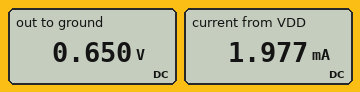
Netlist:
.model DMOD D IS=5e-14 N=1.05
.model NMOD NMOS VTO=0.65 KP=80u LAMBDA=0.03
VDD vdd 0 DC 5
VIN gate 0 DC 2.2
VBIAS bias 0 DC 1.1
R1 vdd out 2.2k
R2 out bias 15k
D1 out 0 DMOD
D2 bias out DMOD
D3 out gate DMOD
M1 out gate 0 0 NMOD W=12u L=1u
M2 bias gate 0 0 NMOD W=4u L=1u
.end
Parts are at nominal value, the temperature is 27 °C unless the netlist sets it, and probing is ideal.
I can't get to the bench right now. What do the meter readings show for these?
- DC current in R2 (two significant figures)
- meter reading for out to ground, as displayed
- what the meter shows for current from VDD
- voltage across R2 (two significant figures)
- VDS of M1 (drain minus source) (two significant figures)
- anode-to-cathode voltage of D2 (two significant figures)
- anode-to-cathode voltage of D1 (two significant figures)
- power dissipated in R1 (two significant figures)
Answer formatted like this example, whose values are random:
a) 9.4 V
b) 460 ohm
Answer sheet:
a) 30 µA
b) 0.650 V
c) 1.977 mA
d) 450 mV
e) 650 mV
f) 450 mV
g) 650 mV
h) 8.6 mW
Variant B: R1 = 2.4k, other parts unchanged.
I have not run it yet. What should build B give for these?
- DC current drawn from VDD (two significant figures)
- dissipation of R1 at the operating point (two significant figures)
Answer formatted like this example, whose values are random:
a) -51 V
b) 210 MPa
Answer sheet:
a) 1.8 mA
b) 7.9 mW
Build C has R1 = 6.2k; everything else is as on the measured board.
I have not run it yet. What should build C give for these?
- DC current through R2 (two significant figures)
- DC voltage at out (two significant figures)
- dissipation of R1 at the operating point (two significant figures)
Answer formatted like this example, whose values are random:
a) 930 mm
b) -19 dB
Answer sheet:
a) 35 µA
b) 570 mV
c) 3.2 mW
